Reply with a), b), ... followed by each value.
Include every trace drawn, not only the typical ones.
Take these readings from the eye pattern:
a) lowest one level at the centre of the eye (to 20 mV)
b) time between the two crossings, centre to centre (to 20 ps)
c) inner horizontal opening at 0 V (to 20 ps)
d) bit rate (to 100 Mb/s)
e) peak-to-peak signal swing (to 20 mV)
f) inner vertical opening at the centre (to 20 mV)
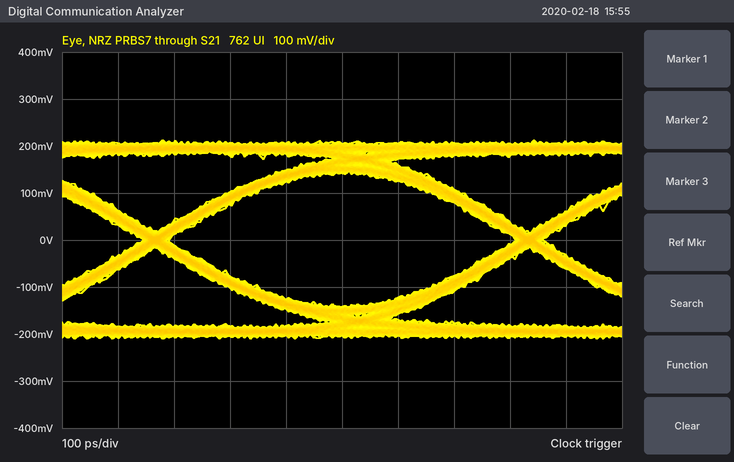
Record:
a) 140 mV
b) 660 ps
c) 620 ps
d) 1.5 Gb/s
e) 420 mV
f) 280 mV
